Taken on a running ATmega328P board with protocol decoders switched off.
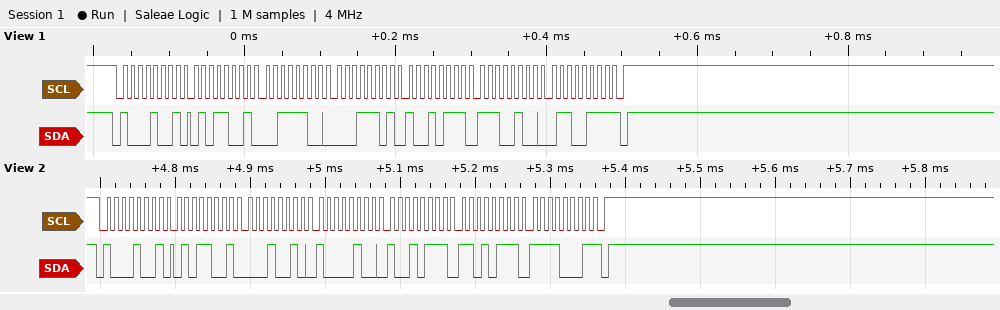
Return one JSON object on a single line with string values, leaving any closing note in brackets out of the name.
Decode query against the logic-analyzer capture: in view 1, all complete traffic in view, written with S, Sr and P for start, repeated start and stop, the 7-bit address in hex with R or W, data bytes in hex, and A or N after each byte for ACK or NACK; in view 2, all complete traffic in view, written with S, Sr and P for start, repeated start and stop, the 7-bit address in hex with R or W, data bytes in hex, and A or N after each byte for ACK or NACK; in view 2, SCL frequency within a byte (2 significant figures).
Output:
{"in view 1, all complete traffic in view, written with S, Sr and P for start, repeated start and stop, the 7-bit address in hex with R or W, data bytes in hex, and A or N after each byte for ACK or NACK": "S 44R A 59 A 3C A 1D A 97 A E4 A 67 N P", "in view 2, all complete traffic in view, written with S, Sr and P for start, repeated start and stop, the 7-bit address in hex with R or W, data bytes in hex, and A or N after each byte for ACK or NACK": "S 44R A 59 A 12 A 84 A 97 A D7 A F1 N P", "in view 2, SCL frequency within a byte": "100 kHz"}
